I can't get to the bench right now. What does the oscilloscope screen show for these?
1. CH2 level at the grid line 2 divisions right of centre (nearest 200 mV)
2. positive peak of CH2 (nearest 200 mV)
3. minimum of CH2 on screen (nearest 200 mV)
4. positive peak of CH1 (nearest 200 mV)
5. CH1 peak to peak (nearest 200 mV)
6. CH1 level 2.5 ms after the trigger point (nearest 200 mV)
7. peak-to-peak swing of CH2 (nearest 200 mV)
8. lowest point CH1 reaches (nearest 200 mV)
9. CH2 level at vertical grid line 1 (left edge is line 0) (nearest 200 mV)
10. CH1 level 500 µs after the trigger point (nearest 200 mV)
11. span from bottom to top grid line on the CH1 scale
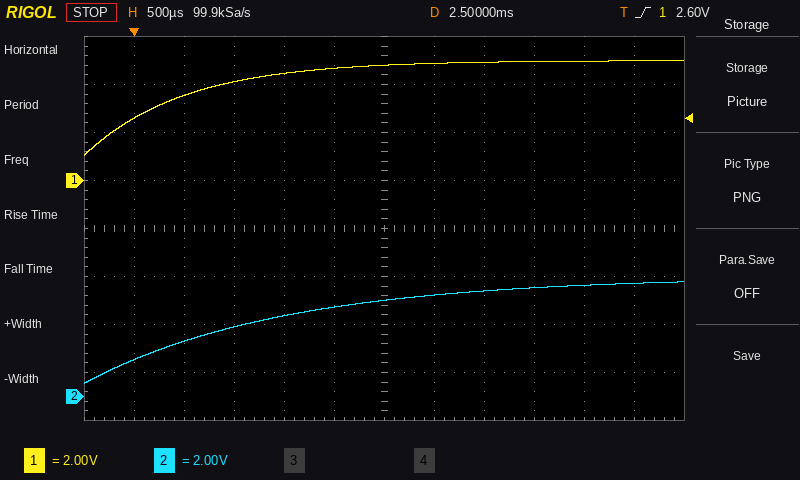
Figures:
4.4 V
4.8 V
600 mV
5.0 V
4.0 V
4.8 V
4.2 V
1.0 V
1.6 V
3.6 V
16 V
